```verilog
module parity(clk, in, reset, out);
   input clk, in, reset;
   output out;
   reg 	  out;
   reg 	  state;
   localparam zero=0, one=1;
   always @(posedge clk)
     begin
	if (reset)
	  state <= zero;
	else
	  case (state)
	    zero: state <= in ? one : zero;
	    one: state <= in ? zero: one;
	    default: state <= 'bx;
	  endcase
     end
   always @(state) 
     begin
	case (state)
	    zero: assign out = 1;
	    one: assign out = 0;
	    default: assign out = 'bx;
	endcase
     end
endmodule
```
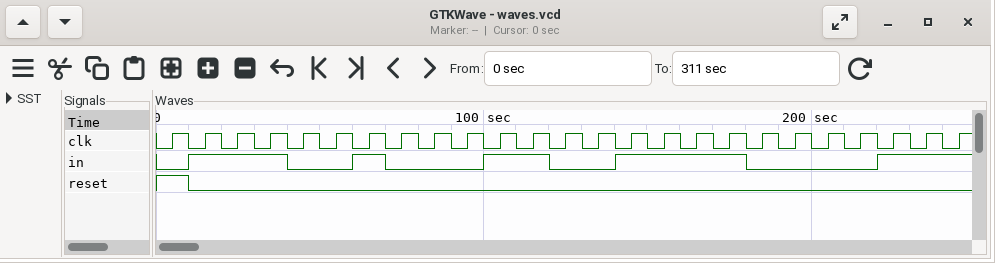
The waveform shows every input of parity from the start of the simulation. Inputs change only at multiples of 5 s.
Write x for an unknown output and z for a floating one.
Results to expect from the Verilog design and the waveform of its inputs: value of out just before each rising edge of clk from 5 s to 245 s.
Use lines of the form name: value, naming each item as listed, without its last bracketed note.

value of out just before each rising edge of clk from 5 s to 245 s: x 1 0 1 0 0 0 1 1 1 1 0 1 1 1 0 1 0 1 1 1 1 1 0 1
